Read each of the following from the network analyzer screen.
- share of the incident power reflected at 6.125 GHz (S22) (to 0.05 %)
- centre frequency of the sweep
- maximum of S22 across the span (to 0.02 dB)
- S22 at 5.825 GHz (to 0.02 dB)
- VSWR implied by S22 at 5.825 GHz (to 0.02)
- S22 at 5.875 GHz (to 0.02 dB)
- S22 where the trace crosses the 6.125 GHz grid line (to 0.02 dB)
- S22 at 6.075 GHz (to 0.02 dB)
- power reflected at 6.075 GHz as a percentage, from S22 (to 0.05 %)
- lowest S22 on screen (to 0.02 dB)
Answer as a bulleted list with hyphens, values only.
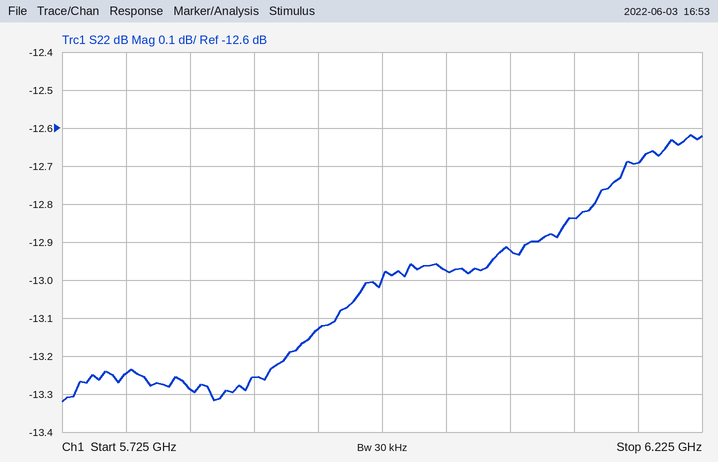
- 5.20 %
- 5.975 GHz
- -12.62 dB
- -13.28 dB
- 1.56
- -13.26 dB
- -12.84 dB
- -12.92 dB
- 5.10 %
- -13.32 dB
